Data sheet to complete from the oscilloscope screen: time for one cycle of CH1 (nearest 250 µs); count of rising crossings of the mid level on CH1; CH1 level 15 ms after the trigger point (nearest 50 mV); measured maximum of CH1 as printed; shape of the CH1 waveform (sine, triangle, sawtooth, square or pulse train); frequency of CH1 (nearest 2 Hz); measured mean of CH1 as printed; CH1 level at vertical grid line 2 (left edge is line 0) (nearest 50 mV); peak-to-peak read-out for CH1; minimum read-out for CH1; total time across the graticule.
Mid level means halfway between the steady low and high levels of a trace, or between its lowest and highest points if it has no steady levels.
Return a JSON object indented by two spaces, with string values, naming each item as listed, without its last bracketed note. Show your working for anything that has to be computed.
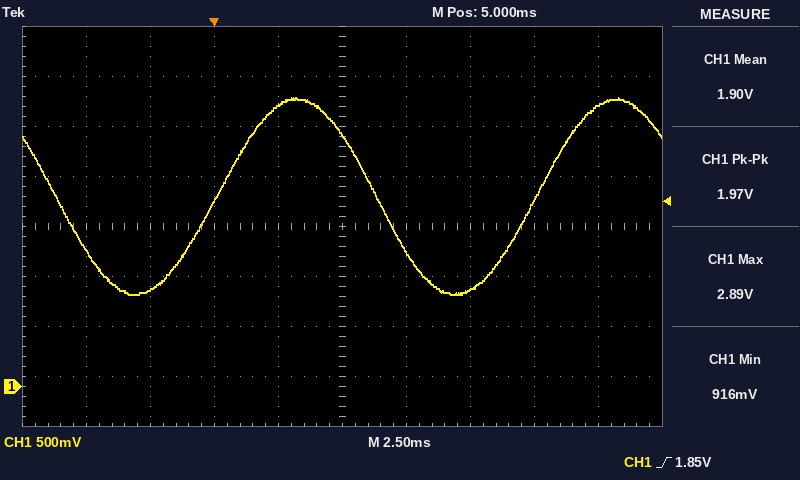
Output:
{
  "time for one cycle of CH1": "12.50 ms",
  "count of rising crossings of the mid level on CH1": "2",
  "CH1 level 15 ms after the trigger point": "2.80 V",
  "measured maximum of CH1 as printed": "2.89 V",
  "shape of the CH1 waveform": "sine",
  "frequency of CH1": "1 / 12.50 ms ≈ 80 Hz",
  "measured mean of CH1 as printed": "1.90 V",
  "CH1 level at vertical grid line 2 (left edge is line 0)": "950 mV",
  "peak-to-peak read-out for CH1": "1.97 V",
  "minimum read-out for CH1": "916 mV",
  "total time across the graticule": "25 ms"
}
